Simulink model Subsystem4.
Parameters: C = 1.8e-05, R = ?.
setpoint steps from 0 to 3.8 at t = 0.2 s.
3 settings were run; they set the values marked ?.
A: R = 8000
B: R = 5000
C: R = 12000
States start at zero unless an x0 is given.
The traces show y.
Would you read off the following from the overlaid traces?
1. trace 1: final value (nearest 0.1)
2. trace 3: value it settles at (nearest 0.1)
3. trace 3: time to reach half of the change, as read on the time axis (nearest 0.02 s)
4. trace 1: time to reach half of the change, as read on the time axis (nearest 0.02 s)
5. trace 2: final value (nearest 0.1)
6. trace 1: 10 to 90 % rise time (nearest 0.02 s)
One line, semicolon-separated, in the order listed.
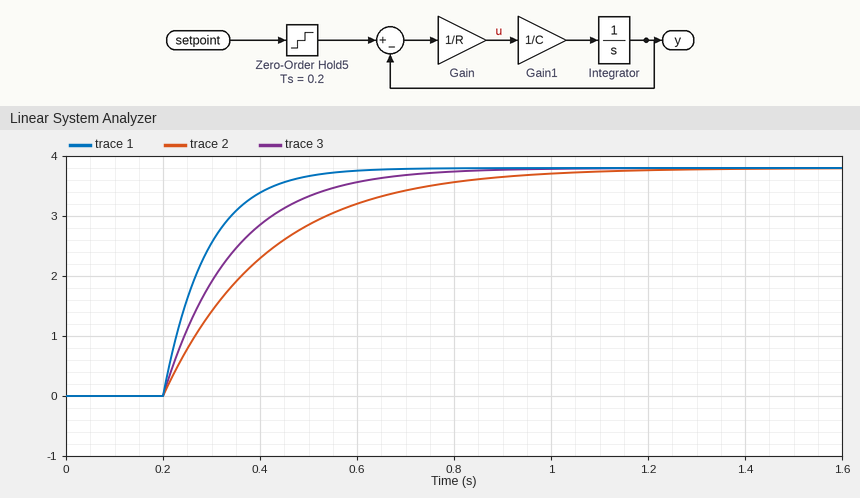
3.8; 3.8; 0.30 s; 0.26 s; 3.8; 0.20 s
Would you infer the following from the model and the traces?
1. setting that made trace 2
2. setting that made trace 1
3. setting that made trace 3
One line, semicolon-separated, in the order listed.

C; B; A
